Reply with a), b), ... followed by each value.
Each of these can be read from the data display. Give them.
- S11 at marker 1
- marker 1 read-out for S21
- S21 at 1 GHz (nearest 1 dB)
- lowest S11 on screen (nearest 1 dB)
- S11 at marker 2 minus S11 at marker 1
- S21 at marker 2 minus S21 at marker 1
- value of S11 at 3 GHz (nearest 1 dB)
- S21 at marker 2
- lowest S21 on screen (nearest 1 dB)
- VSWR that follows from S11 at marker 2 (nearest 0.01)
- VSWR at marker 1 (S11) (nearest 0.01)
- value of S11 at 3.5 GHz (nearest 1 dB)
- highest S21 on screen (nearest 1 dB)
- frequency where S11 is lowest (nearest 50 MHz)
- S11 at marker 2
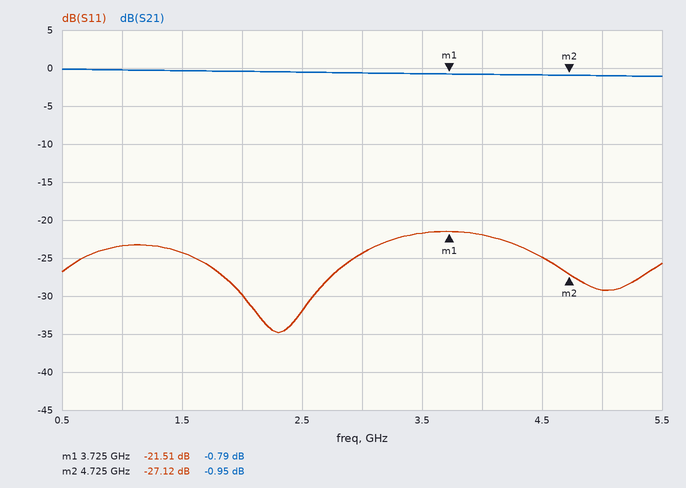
a) -21.51 dB
b) -0.79 dB
c) 0 dB
d) -35 dB
e) -5.61 dB
f) -0.16 dB
g) -24 dB
h) -0.95 dB
i) -1 dB
j) 1.09
k) 1.18
l) -22 dB
m) 0 dB
n) 2.30 GHz
o) -27.12 dB
